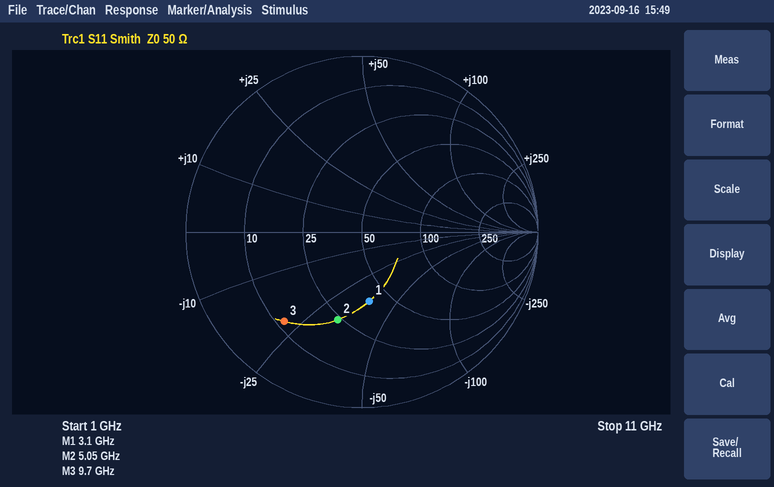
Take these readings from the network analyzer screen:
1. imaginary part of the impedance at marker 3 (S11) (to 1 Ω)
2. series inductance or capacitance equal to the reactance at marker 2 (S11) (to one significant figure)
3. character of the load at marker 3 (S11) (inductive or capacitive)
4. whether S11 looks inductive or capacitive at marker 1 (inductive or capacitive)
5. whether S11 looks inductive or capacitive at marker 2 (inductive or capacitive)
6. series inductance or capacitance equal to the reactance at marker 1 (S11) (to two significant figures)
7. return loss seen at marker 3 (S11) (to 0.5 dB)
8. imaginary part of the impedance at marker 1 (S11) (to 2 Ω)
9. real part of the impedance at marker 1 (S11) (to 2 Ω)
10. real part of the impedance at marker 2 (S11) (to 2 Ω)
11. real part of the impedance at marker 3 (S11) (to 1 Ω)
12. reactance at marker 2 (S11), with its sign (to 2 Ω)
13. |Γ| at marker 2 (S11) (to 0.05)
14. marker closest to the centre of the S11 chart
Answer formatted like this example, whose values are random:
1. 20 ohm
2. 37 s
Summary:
1. -22 Ω
2. 1.0 pF
3. capacitive
4. capacitive
5. capacitive
6. 1.4 pF
7. 3.5 dB
8. -36 Ω
9. 40 Ω
10. 24 Ω
11. 12 Ω
12. -32 Ω
13. 0.50
14. marker 1
